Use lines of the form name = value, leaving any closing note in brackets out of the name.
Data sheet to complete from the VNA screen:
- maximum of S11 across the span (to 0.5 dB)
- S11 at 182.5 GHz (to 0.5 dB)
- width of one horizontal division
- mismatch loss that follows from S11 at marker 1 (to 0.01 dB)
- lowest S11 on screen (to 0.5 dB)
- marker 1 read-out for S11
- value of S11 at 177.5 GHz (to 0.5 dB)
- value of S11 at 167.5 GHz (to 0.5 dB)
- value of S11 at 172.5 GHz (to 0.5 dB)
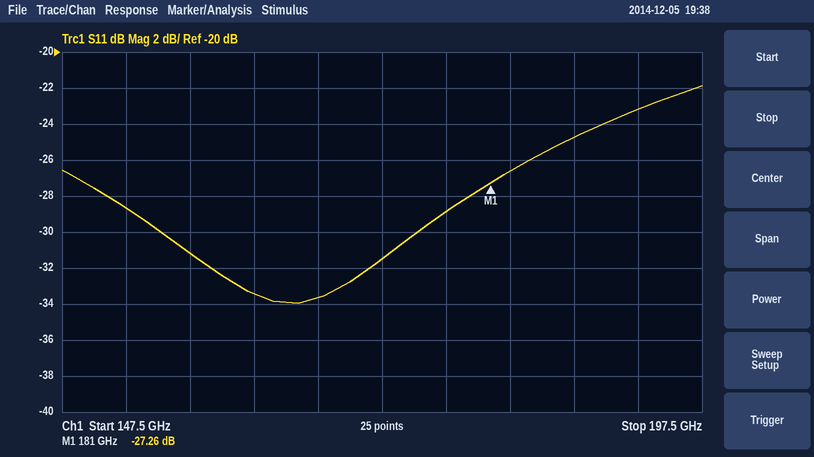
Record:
maximum of S11 across the span = -22.0 dB
S11 at 182.5 GHz = -26.5 dB
width of one horizontal division = 5 GHz
mismatch loss that follows from S11 at marker 1 = 0.01 dB
lowest S11 on screen = -34.0 dB
marker 1 read-out for S11 = -27.26 dB
value of S11 at 177.5 GHz = -29.0 dB
value of S11 at 167.5 GHz = -33.5 dB
value of S11 at 172.5 GHz = -31.5 dB
